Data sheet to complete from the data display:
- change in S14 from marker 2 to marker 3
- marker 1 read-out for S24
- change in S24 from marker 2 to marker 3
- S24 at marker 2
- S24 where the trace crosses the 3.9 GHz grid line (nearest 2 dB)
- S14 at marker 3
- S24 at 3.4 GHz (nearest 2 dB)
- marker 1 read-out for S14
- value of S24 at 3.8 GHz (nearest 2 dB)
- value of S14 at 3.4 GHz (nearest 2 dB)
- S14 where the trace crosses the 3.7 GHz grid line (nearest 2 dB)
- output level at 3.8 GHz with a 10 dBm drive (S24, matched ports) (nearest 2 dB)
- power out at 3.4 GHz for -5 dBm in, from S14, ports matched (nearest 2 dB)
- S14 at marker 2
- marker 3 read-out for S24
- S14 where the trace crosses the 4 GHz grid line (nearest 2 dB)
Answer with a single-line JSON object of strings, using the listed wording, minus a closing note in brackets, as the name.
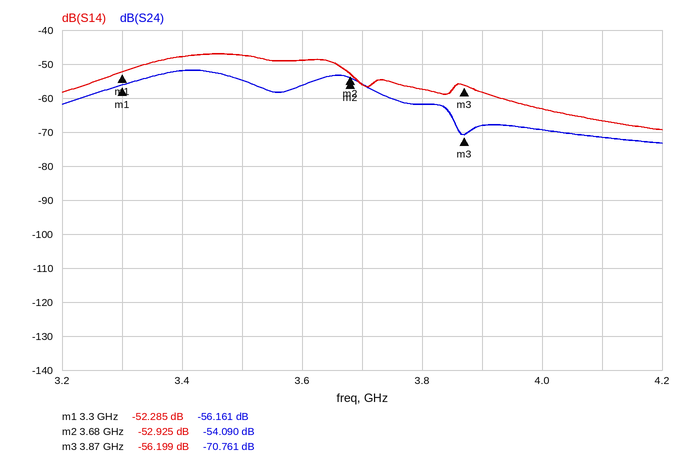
{"change in S14 from marker 2 to marker 3": "-3.274 dB", "marker 1 read-out for S24": "-56.161 dB", "change in S24 from marker 2 to marker 3": "-16.671 dB", "S24 at marker 2": "-54.090 dB", "S24 where the trace crosses the 3.9 GHz grid line": "-68 dB", "S14 at marker 3": "-56.199 dB", "S24 at 3.4 GHz": "-52 dB", "marker 1 read-out for S14": "-52.285 dB", "value of S24 at 3.8 GHz": "-62 dB", "value of S14 at 3.4 GHz": "-48 dB", "S14 where the trace crosses the 3.7 GHz grid line": "-56 dB", "output level at 3.8 GHz with a 10 dBm drive (S24, matched ports)": "-52 dBm", "power out at 3.4 GHz for -5 dBm in, from S14, ports matched": "-52 dBm", "S14 at marker 2": "-52.925 dB", "marker 3 read-out for S24": "-70.761 dB", "S14 where the trace crosses the 4 GHz grid line": "-64 dB"}
